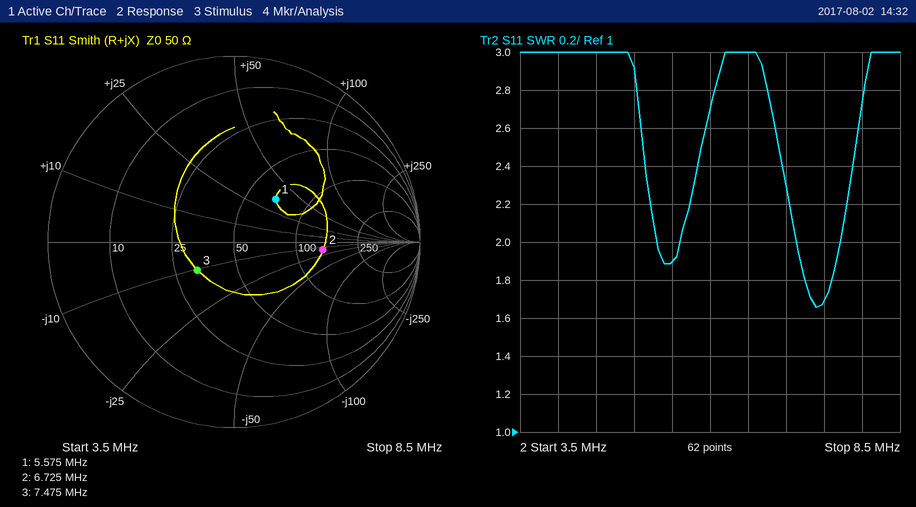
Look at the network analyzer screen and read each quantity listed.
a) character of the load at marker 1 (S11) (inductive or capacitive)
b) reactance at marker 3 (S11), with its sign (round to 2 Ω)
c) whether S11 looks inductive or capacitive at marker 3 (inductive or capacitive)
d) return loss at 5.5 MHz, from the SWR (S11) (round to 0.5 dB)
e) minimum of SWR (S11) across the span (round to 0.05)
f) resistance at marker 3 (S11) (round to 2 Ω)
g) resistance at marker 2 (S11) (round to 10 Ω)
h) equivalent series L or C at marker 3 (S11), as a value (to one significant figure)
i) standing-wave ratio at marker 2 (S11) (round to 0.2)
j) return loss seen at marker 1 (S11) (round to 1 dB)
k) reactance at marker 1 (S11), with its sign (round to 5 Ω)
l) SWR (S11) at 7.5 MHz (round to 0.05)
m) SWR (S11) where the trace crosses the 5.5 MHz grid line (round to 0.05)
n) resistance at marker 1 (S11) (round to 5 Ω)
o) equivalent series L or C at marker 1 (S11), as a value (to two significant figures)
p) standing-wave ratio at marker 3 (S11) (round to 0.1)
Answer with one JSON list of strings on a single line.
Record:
["inductive", "-10 Ω", "capacitive", "10.0 dB", "1.65", "32 Ω", "140 Ω", "2 nF", "2.8", "10 dB", "+35 Ω", "1.70", "1.90", "70 Ω", "1.0 µH", "1.7"]
